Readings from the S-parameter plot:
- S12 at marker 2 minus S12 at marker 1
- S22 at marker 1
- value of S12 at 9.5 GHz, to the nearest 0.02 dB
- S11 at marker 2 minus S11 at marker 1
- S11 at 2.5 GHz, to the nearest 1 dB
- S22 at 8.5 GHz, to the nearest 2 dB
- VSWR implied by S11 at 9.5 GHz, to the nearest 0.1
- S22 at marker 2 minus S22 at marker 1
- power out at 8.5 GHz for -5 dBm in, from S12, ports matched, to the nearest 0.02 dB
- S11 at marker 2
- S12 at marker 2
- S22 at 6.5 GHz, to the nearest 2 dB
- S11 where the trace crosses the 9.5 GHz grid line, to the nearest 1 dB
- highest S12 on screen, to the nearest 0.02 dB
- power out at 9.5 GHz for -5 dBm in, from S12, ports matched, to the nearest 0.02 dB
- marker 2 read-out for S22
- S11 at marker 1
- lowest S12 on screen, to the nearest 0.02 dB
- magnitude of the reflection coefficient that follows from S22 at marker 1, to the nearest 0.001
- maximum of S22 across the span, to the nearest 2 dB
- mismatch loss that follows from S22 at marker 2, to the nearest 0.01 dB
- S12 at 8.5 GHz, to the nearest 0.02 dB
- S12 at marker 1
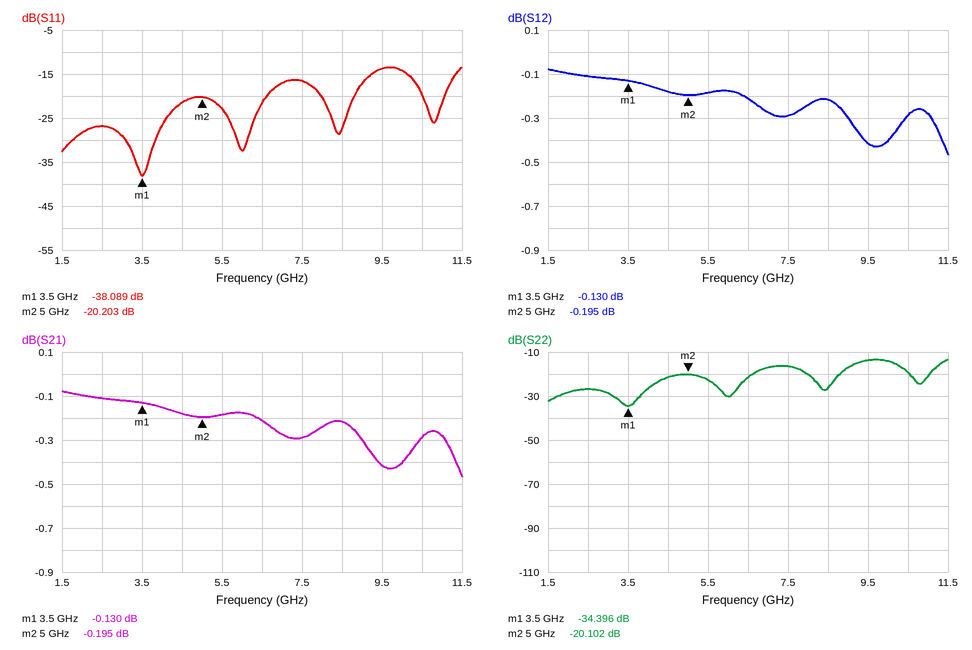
-0.065 dB
-34.396 dB
-0.42 dB
17.886 dB
-27 dB
-26 dB
1.5
14.294 dB
-5.22 dBm
-20.203 dB
-0.195 dB
-22 dB
-14 dB
-0.08 dB
-5.42 dBm
-20.102 dB
-38.089 dB
-0.46 dB
0.019
-14 dB
0.04 dB
-0.22 dB
-0.130 dB
